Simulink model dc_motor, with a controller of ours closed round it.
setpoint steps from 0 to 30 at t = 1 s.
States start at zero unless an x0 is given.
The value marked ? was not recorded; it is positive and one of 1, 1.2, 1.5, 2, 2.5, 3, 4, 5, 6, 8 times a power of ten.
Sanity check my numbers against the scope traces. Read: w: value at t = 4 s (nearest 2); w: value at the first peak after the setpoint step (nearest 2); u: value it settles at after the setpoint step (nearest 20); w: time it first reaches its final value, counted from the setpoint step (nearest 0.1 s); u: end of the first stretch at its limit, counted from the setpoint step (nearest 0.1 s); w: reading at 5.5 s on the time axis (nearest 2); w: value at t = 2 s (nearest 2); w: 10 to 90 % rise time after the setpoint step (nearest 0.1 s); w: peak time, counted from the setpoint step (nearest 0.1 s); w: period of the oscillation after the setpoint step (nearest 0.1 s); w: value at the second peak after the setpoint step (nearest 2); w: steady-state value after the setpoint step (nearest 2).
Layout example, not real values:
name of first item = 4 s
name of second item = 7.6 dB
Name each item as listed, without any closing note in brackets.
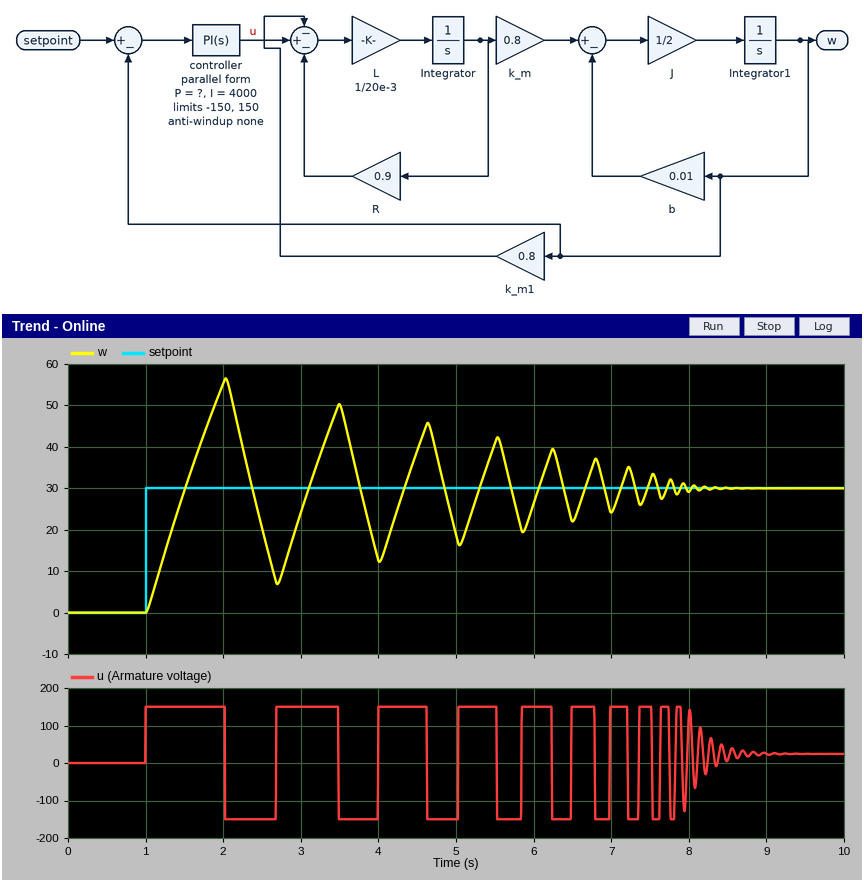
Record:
w: value at t = 4 s = 12
w: value at the first peak after the setpoint step = 56
u: value it settles at after the setpoint step = 20
w: time it first reaches its final value, counted from the setpoint step = 0.5 s
u: end of the first stretch at its limit, counted from the setpoint step = 1.0 s
w: reading at 5.5 s on the time axis = 40
w: value at t = 2 s = 56
w: 10 to 90 % rise time after the setpoint step = 0.4 s
w: peak time, counted from the setpoint step = 1.0 s
w: period of the oscillation after the setpoint step = 1.5 s
w: value at the second peak after the setpoint step = 50
w: steady-state value after the setpoint step = 30
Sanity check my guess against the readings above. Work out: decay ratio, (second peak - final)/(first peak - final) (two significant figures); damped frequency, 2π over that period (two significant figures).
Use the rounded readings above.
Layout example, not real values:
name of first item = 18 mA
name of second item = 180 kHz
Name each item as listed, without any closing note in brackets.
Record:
decay ratio, (second peak - final)/(first peak - final) = 0.77
damped frequency, 2π over that period = 4.2 rad/s
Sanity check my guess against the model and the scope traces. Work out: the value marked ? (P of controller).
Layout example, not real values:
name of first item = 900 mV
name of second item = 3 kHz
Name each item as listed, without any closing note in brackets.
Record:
the value marked ? = 120
